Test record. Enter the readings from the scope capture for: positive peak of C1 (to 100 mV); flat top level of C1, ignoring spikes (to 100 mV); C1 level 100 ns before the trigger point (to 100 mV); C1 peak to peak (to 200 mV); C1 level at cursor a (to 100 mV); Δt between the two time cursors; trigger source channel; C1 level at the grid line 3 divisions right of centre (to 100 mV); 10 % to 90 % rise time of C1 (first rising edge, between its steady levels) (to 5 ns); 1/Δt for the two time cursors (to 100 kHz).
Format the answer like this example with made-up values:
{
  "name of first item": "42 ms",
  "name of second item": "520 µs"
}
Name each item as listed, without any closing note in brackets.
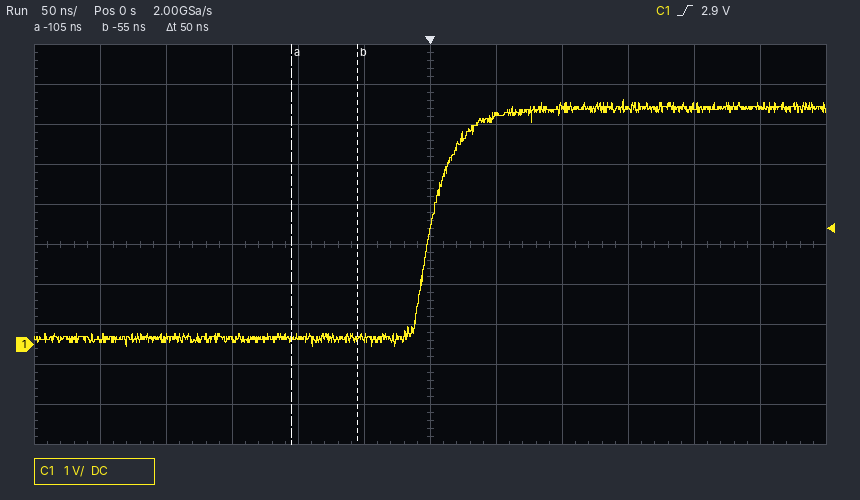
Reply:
{
  "positive peak of C1": "6.1 V",
  "flat top level of C1, ignoring spikes": "5.9 V",
  "C1 level 100 ns before the trigger point": "200 mV",
  "C1 peak to peak": "6.2 V",
  "C1 level at cursor a": "100 mV",
  "Δt between the two time cursors": "50 ns",
  "trigger source channel": "C1",
  "C1 level at the grid line 3 divisions right of centre": "5.9 V",
  "10 % to 90 % rise time of C1 (first rising edge, between its steady levels)": "40 ns",
  "1/Δt for the two time cursors": "20.0 MHz"
}
